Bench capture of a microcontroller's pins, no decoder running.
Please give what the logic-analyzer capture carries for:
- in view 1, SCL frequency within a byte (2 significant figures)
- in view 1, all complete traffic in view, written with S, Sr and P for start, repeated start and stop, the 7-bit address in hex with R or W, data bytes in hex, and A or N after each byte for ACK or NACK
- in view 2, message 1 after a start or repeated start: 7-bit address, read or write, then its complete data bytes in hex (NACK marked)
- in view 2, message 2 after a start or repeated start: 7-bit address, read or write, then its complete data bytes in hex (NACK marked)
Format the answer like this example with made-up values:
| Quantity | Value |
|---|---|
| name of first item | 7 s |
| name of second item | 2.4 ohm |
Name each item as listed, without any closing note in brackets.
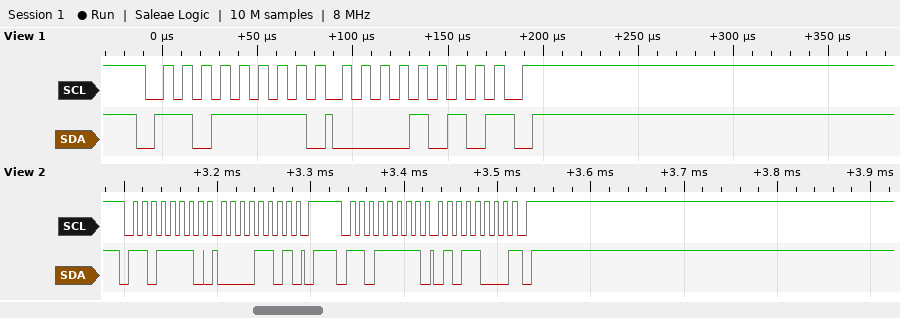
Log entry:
| Quantity | Value |
|---|---|
| in view 1, SCL frequency within a byte | 100 kHz |
| in view 1, all complete traffic in view, written with S, Sr and P for start, repeated start and stop, the 7-bit address in hex with R or W, data bytes in hex, and A or N after each byte for ACK or NACK | S 6FR A 0A N P |
| in view 2, message 1 after a start or repeated start: 7-bit address, read or write, then its complete data bytes in hex | 0x6F write: 0D |
| in view 2, message 2 after a start or repeated start: 7-bit address, read or write, then its complete data bytes in hex | 0x6F read: 58 NACK |
